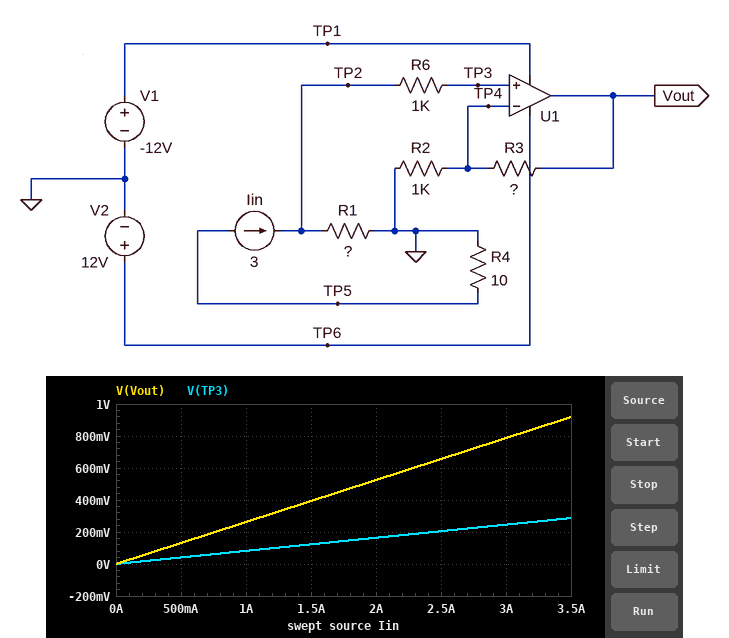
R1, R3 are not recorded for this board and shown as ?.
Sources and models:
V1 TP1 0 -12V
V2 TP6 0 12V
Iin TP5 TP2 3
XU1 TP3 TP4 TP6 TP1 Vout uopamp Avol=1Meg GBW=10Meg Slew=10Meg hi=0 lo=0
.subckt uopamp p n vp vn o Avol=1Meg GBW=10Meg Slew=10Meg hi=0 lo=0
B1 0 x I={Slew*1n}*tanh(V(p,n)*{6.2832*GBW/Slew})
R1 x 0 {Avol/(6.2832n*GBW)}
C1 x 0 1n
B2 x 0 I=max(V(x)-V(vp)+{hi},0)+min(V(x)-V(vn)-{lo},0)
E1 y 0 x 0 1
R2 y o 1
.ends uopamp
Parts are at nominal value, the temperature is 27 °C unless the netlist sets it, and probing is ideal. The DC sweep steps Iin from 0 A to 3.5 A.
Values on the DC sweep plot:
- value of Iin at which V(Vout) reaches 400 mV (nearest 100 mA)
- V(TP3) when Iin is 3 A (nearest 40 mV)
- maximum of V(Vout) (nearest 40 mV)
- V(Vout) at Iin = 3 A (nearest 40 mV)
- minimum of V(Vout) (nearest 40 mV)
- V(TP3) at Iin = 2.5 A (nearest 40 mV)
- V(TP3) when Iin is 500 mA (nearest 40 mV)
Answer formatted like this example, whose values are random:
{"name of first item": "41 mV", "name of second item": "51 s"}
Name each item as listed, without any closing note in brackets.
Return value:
{"value of Iin at which V(Vout) reaches 400 mV": "1.5 A", "V(TP3) when Iin is 3 A": "240 mV", "maximum of V(Vout)": "920 mV", "V(Vout) at Iin = 3 A": "800 mV", "minimum of V(Vout)": "0 V", "V(TP3) at Iin = 2.5 A": "200 mV", "V(TP3) when Iin is 500 mA": "40 mV"}
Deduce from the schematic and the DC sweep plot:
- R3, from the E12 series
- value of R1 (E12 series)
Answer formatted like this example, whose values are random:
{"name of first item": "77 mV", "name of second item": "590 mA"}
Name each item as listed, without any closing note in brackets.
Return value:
{"R3, from the E12 series": "2.2 kΩ", "value of R1": "0.082 Ω"}
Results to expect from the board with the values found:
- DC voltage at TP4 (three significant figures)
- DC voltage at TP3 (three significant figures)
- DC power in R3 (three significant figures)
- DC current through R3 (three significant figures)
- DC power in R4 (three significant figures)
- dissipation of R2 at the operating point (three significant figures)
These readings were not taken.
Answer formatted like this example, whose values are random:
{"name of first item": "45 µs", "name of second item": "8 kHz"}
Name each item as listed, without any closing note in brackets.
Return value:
{"DC voltage at TP4": "246 mV", "DC voltage at TP3": "246 mV", "DC power in R3": "133 µW", "DC current through R3": "246 µA", "DC power in R4": "90.0 W", "dissipation of R2 at the operating point": "60.5 µW"}
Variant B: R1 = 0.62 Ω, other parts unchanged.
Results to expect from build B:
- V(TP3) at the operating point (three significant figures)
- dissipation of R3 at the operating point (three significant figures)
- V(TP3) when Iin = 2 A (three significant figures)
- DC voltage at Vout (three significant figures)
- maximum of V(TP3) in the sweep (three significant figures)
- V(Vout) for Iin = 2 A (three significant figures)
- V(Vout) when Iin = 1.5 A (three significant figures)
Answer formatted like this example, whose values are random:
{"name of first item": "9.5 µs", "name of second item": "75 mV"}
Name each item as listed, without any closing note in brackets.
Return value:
{"V(TP3) at the operating point": "1.86 V", "dissipation of R3 at the operating point": "7.61 mW", "V(TP3) when Iin = 2 A": "1.24 V", "DC voltage at Vout": "5.95 V", "maximum of V(TP3) in the sweep": "2.17 V", "V(Vout) for Iin = 2 A": "3.97 V", "V(Vout) when Iin = 1.5 A": "2.98 V"}
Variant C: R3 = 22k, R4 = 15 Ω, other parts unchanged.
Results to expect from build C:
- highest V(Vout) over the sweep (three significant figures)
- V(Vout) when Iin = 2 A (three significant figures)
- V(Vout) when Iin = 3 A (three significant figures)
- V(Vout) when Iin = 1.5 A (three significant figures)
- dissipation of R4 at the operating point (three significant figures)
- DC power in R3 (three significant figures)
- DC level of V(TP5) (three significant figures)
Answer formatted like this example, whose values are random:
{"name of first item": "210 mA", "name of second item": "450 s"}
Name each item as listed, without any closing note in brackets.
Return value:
{"highest V(Vout) over the sweep": "6.60 V", "V(Vout) when Iin = 2 A": "3.77 V", "V(Vout) when Iin = 3 A": "5.66 V", "V(Vout) when Iin = 1.5 A": "2.83 V", "dissipation of R4 at the operating point": "135 W", "DC power in R3": "1.33 mW", "DC level of V(TP5)": "-45.0 V"}
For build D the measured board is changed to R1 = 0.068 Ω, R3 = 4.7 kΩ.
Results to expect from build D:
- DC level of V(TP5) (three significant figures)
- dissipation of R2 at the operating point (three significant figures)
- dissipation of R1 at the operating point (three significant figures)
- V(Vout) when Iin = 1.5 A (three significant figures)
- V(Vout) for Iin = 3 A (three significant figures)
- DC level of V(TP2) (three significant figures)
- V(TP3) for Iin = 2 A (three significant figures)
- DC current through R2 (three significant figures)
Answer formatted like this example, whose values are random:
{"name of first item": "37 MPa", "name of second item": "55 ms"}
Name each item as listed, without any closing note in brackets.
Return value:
{"DC level of V(TP5)": "-30.0 V", "dissipation of R2 at the operating point": "41.6 µW", "dissipation of R1 at the operating point": "612 mW", "V(Vout) when Iin = 1.5 A": "581 mV", "V(Vout) for Iin = 3 A": "1.16 V", "DC level of V(TP2)": "204 mV", "V(TP3) for Iin = 2 A": "136 mV", "DC current through R2": "204 µA"}
